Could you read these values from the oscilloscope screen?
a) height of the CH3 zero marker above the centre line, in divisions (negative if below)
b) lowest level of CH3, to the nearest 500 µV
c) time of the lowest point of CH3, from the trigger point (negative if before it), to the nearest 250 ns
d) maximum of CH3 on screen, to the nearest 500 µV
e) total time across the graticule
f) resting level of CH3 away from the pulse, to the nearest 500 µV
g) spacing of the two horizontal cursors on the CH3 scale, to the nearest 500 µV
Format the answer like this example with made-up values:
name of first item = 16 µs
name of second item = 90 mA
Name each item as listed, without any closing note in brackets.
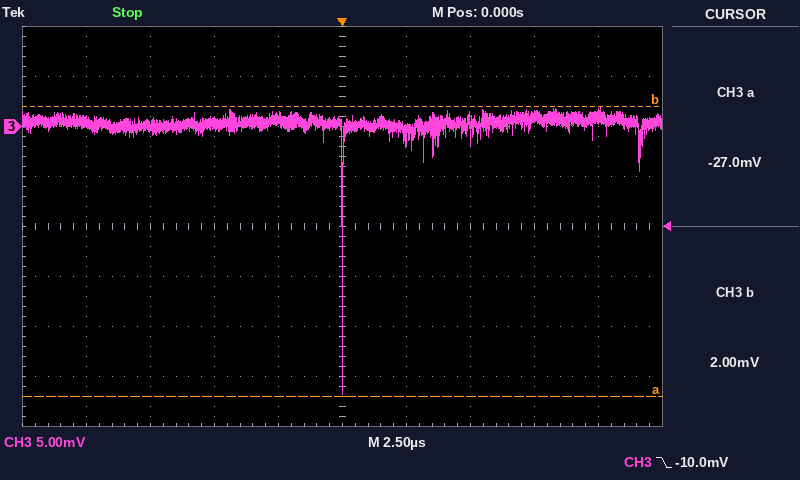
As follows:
height of the CH3 zero marker above the centre line, in divisions = +2.0 div
lowest level of CH3, to the nearest 500 µV = -27.0 mV
time of the lowest point of CH3, from the trigger point (negative if before it), to the nearest 250 ns = 0.00 µs
maximum of CH3 on screen, to the nearest 500 µV = 2.0 mV
total time across the graticule = 25 µs
resting level of CH3 away from the pulse, to the nearest 500 µV = 500 µV
spacing of the two horizontal cursors on the CH3 scale, to the nearest 500 µV = 29.0 mV
